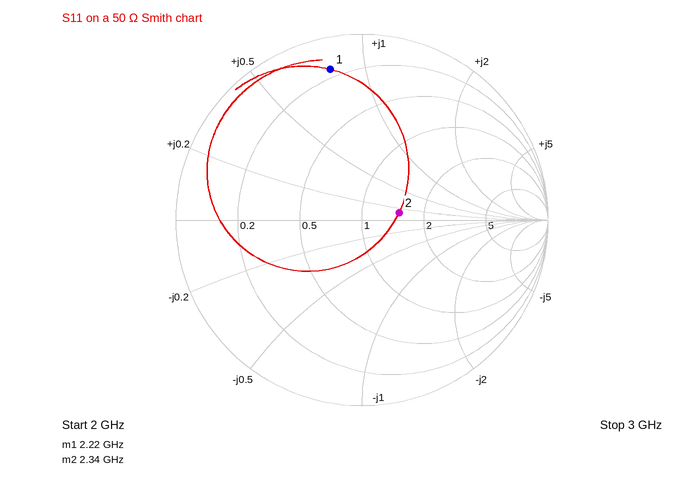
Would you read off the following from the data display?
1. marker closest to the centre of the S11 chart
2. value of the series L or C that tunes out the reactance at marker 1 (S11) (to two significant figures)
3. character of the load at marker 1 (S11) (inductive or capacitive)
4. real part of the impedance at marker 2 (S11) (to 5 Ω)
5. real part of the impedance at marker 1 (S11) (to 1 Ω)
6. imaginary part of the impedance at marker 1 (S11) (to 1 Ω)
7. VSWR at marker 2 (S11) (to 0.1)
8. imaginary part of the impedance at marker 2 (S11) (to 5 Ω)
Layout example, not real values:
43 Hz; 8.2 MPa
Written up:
marker 2; 1.8 pF; inductive; 75 Ω; 8 Ω; +40 Ω; 1.5; +5 Ω
